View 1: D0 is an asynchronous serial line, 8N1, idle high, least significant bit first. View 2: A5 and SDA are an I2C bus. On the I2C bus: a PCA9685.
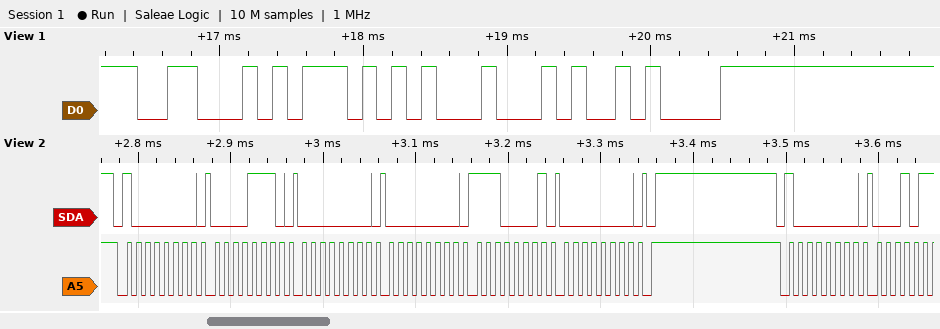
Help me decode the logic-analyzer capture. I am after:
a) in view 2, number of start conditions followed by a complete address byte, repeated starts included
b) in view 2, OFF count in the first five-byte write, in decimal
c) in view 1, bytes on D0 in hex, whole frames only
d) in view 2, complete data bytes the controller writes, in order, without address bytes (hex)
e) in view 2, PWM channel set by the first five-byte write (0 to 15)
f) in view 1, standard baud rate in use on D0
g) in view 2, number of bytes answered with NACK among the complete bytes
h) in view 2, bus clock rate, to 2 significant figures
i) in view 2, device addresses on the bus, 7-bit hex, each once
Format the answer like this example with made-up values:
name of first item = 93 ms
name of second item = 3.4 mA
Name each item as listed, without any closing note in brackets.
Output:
in view 2, number of start conditions followed by a complete address byte, repeated starts included = 2
in view 2, OFF count in the first five-byte write, in decimal = 225
in view 1, bytes on D0 in hex, whole frames only = 46 57 44 0A
in view 2, complete data bytes the controller writes, in order, without address bytes = 0E 00 00 E1 00
in view 2, PWM channel set by the first five-byte write = 2
in view 1, standard baud rate in use on D0 = 9600 baud
in view 2, number of bytes answered with NACK among the complete bytes = 0
in view 2, bus clock rate, to 2 significant figures = 100 kHz
in view 2, device addresses on the bus, 7-bit hex, each once = 0x40
